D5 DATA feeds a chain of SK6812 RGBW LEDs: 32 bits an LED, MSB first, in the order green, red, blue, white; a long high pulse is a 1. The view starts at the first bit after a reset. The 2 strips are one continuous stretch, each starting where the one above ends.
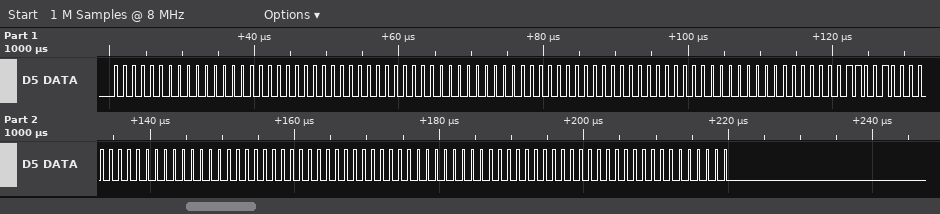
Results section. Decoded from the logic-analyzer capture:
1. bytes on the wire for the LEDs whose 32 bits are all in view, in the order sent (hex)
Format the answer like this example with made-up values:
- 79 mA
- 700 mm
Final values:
- 00 00 00 00 00 00 00 00 00 00 64 00 00 00 00 00 00 00 00 00
